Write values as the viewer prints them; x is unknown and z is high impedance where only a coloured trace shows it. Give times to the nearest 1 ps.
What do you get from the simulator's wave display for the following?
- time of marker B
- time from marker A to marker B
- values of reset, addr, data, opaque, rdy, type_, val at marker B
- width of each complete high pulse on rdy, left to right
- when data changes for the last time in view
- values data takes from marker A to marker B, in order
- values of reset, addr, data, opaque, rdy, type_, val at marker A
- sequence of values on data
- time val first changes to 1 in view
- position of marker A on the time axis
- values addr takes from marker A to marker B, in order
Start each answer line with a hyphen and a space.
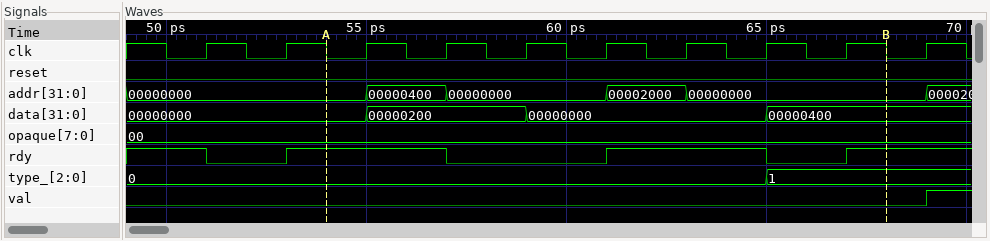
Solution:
- 68 ps
- 14 ps
- reset=0, addr=00000000, data=00000400, opaque=00, rdy=1, type_=1, val=0
- 4 ps, 4 ps
- 65 ps
- 00000000, 00000200, 00000000, 00000400
- reset=0, addr=00000000, data=00000000, opaque=00, rdy=1, type_=0, val=0
- 00000000, 00000200, 00000000, 00000400
- 69 ps
- 54 ps
- 00000000, 00000400, 00000000, 00002000, 00000000
